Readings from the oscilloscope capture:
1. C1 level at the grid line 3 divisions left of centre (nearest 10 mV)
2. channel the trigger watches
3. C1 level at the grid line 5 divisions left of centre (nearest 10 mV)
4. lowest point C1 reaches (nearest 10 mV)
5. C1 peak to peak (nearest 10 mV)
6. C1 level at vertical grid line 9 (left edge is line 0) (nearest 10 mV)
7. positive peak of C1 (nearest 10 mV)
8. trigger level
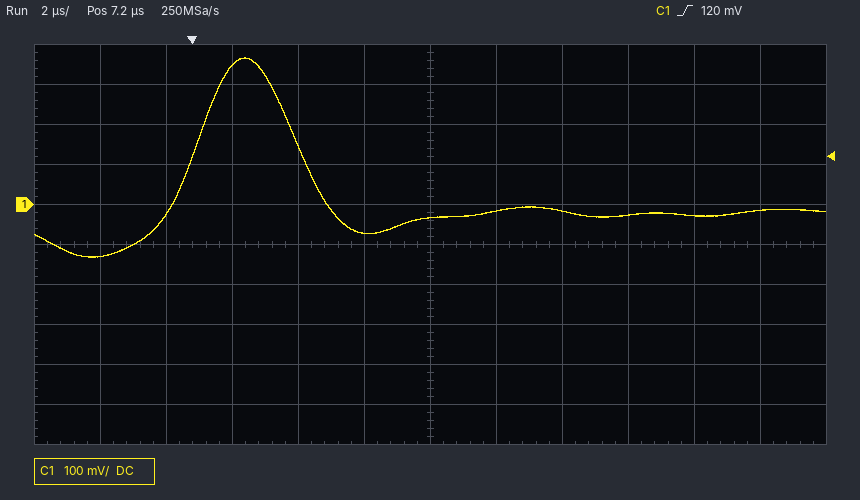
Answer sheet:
350 mV
C1
-130 mV
-130 mV
500 mV
-30 mV
370 mV
120 mV
